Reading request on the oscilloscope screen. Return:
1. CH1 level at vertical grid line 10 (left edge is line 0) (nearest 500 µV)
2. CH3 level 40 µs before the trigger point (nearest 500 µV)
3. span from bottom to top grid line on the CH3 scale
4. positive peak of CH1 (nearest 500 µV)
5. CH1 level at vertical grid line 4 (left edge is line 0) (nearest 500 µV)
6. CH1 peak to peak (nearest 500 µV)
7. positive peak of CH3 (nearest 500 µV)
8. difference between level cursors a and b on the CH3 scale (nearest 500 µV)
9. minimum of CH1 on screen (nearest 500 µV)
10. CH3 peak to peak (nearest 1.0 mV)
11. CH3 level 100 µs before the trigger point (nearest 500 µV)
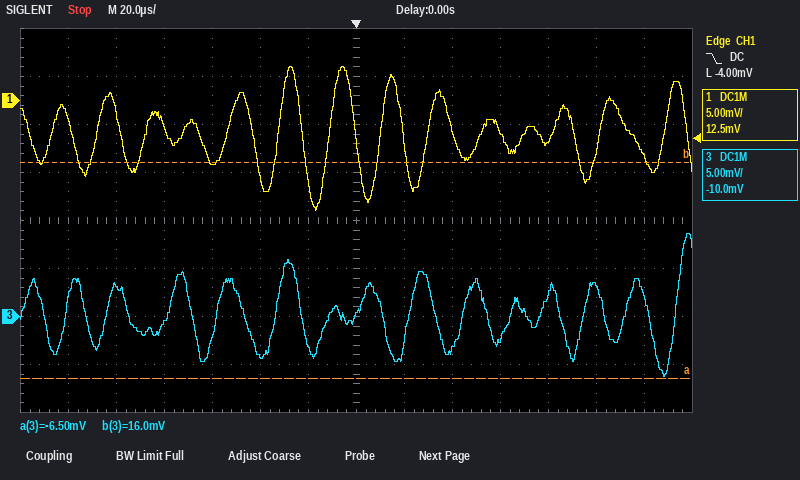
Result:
-3.0 mV
-4.0 mV
40 mV
3.5 mV
-6.5 mV
15.0 mV
8.5 mV
22.5 mV
-11.5 mV
15.0 mV
3.0 mV
